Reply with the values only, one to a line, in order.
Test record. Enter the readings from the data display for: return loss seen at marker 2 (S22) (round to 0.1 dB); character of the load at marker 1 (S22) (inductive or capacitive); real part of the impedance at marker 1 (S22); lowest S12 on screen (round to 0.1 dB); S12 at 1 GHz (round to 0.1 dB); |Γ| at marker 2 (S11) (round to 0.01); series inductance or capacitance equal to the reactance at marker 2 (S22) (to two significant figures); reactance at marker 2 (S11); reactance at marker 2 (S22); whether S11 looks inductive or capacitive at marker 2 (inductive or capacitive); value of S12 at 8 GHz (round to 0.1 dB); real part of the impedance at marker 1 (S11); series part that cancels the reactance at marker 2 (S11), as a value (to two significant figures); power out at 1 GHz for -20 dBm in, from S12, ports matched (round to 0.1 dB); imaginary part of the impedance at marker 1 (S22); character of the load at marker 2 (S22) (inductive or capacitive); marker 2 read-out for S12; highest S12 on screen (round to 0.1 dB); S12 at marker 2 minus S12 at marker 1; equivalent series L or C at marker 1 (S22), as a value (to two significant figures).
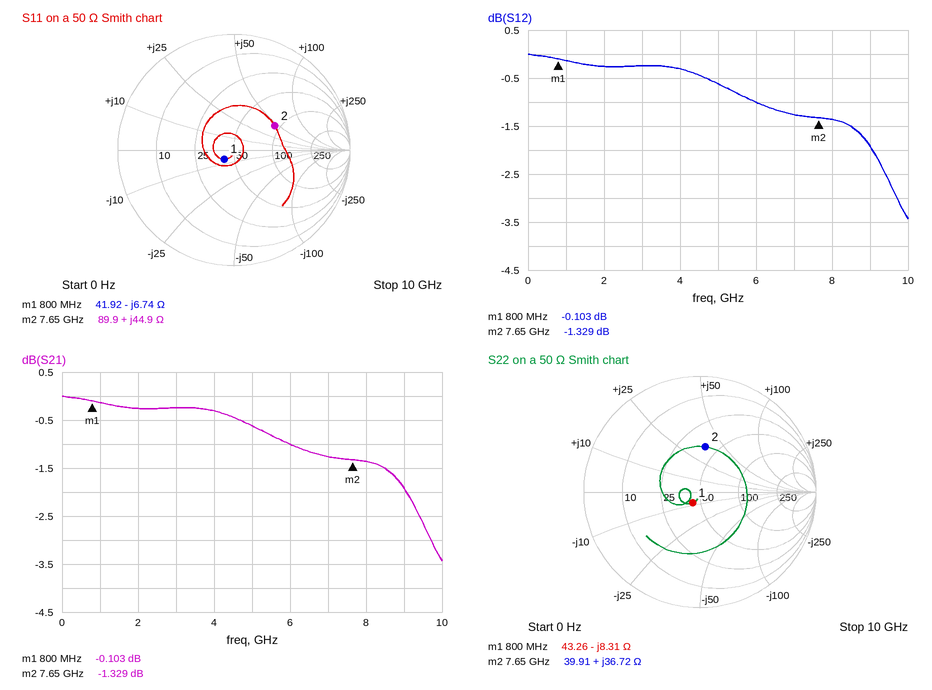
8.1 dB
capacitive
43.26 Ω
-3.4 dB
-0.1 dB
0.41
760 pH
+44.9 Ω
+36.72 Ω
inductive
-1.4 dB
41.92 Ω
460 fF
-20.1 dBm
-8.31 Ω
inductive
-1.329 dB
0.0 dB
-1.226 dB
24 pF
